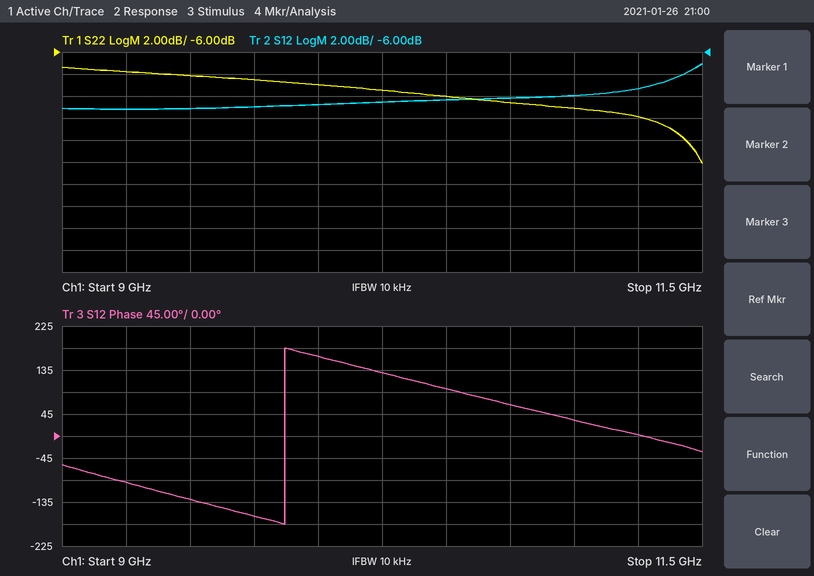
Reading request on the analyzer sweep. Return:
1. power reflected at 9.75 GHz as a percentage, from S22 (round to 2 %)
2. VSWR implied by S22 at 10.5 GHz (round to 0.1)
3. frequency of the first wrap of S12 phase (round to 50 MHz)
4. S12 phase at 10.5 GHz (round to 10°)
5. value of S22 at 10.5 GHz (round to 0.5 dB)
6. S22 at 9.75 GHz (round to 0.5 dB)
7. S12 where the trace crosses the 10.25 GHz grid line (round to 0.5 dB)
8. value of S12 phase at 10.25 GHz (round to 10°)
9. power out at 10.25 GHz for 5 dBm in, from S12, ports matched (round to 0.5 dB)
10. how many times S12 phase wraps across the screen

14 %
1.9
9.85 GHz
100°
-10.0 dB
-8.5 dB
-10.5 dB
130°
-5.5 dBm
1
